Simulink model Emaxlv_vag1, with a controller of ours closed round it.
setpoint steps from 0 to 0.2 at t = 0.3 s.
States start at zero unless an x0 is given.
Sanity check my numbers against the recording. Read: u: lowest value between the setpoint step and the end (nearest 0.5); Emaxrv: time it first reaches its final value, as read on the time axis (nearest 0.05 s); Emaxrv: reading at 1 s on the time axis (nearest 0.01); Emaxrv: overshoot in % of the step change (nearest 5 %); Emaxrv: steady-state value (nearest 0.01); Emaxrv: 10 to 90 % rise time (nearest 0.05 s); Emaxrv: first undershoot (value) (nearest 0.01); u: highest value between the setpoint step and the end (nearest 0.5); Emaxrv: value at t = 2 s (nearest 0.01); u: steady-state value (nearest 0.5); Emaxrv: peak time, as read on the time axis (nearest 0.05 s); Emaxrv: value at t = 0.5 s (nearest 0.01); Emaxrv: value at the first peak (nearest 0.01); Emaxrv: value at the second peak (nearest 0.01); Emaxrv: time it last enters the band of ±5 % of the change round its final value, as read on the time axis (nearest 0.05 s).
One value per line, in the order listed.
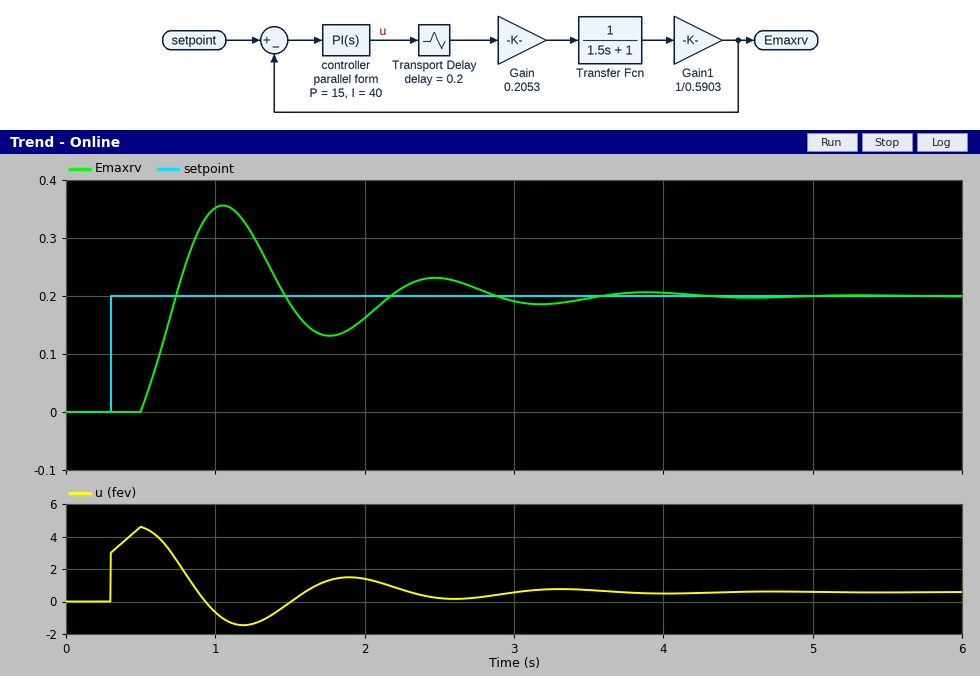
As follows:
-1.5
0.75 s
0.35
80 %
0.20
0.20 s
0.13
4.5
0.16
0.5
1.05 s
0.00
0.36
0.23
3.35 s
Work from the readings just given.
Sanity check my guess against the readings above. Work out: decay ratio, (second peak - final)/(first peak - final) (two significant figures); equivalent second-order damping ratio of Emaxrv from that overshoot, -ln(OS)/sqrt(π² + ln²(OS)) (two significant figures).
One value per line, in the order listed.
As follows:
0.19
0.071
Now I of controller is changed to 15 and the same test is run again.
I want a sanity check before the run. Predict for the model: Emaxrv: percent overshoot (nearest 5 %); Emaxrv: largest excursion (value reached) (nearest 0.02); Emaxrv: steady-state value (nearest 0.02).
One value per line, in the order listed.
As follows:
30 %
0.26
0.20
